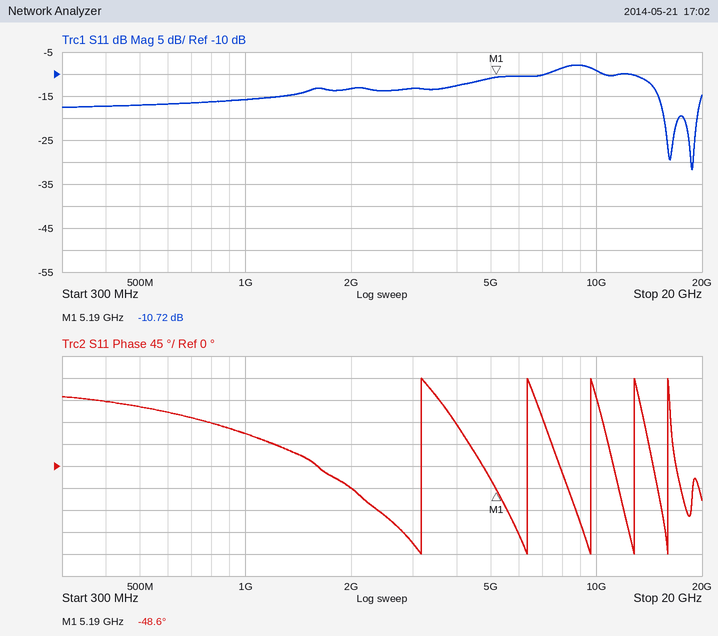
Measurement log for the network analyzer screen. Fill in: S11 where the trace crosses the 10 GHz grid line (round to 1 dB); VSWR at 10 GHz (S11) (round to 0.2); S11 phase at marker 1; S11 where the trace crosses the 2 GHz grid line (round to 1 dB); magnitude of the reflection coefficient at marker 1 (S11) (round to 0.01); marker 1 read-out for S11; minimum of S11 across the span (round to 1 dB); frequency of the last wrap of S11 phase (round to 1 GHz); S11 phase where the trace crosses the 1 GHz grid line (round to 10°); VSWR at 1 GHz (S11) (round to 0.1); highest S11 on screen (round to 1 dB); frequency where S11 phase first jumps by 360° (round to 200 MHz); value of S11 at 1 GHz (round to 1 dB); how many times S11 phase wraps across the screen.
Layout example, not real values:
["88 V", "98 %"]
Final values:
["-9 dB", "2.0", "-48.6°", "-13 dB", "0.29", "-10.72 dB", "-32 dB", "16 GHz", "70°", "1.4", "-8 dB", "3.2 GHz", "-16 dB", "5"]
